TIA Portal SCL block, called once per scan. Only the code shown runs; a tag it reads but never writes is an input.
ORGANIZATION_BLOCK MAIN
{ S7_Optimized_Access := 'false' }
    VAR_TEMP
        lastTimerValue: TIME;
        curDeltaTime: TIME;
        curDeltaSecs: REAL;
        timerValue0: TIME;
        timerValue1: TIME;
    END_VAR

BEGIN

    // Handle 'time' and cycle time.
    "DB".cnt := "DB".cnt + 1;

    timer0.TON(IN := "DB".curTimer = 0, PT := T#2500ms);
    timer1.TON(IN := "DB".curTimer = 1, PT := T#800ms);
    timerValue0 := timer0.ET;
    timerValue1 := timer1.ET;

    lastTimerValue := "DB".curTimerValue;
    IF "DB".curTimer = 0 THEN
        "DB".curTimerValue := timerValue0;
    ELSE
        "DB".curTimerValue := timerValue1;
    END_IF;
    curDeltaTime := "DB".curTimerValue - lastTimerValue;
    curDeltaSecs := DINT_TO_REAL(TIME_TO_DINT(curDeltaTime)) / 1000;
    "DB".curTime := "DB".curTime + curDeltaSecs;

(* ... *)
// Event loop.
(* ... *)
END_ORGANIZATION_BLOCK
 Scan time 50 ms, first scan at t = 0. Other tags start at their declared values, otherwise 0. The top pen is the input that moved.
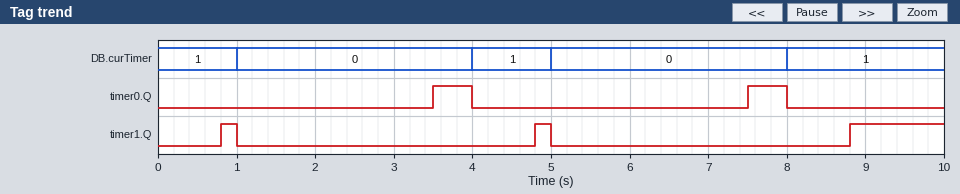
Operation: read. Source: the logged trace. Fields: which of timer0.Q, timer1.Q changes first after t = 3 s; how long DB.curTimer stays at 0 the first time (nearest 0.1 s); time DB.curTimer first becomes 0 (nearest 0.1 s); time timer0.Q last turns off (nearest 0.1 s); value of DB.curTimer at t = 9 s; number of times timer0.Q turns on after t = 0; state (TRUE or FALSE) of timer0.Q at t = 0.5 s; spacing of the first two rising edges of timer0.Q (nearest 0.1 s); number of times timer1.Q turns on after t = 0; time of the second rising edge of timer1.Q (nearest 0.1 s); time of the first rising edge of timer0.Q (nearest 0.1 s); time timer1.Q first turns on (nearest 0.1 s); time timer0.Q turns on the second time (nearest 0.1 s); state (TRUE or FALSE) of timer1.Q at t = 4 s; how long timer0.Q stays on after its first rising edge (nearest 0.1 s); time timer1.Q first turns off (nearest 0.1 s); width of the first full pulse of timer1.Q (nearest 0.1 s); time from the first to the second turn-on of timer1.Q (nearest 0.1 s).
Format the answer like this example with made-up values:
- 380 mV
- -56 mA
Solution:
- timer0.Q
- 3.0 s
- 1.0 s
- 8.0 s
- 1
- 2
- FALSE
- 4.0 s
- 3
- 4.8 s
- 3.5 s
- 0.8 s
- 7.5 s
- FALSE
- 0.5 s
- 1.0 s
- 0.2 s
- 4.0 s
